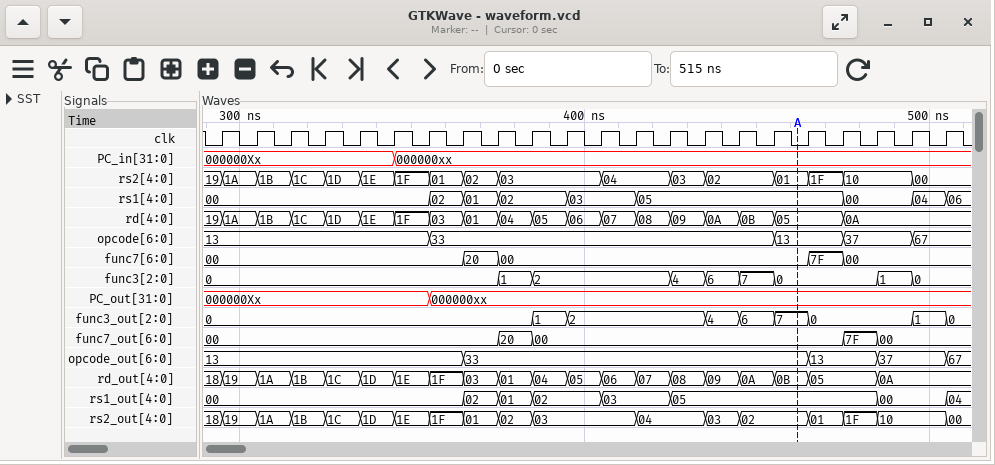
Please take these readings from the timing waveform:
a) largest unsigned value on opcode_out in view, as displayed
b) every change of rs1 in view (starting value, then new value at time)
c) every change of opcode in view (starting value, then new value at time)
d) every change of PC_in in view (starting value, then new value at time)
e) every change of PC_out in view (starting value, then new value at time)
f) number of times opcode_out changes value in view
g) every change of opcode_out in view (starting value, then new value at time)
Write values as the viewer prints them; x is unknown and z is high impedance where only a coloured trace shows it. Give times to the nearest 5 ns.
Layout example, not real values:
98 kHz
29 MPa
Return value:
67
00, 02 at 355 ns, 01 at 365 ns, 02 at 375 ns, 03 at 395 ns, 05 at 415 ns, 00 at 475 ns, 04 at 495 ns, 06 at 505 ns
13, 33 at 355 ns, 13 at 455 ns, 37 at 475 ns, 67 at 495 ns
000000Xx, 000000xx at 345 ns
000000Xx, 000000xx at 355 ns
4
13, 33 at 365 ns, 13 at 465 ns, 37 at 485 ns, 67 at 505 ns
